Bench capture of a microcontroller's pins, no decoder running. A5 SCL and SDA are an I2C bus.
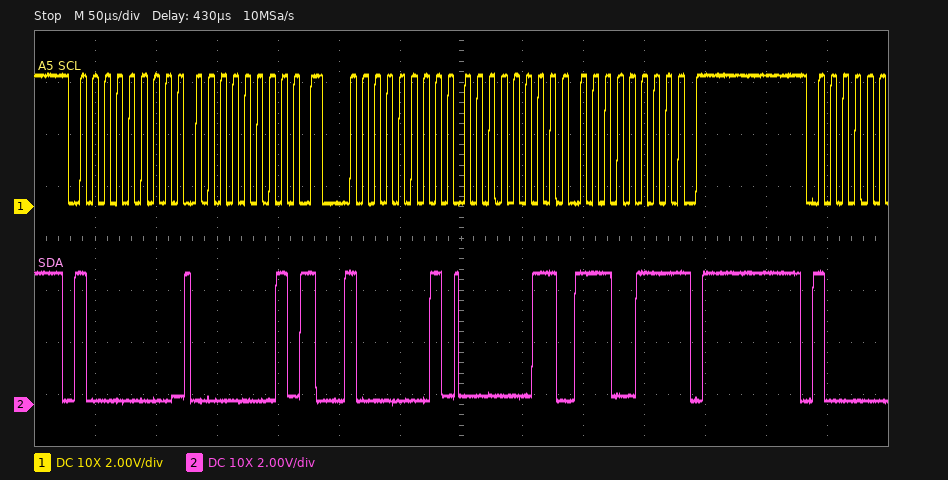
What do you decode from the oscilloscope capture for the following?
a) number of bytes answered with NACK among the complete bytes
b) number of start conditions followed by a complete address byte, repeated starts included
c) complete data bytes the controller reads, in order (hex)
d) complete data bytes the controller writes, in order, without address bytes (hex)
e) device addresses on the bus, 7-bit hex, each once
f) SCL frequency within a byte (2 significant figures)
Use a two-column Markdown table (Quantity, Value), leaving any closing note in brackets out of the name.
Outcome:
| Quantity | Value |
|---|---|
| number of bytes answered with NACK among the complete bytes | 1 |
| number of start conditions followed by a complete address byte, repeated starts included | 2 |
| complete data bytes the controller reads, in order | 03 E7 |
| complete data bytes the controller writes, in order, without address bytes | 01 |
| device addresses on the bus, 7-bit hex, each once | 0x40 |
| SCL frequency within a byte | 100 kHz |
